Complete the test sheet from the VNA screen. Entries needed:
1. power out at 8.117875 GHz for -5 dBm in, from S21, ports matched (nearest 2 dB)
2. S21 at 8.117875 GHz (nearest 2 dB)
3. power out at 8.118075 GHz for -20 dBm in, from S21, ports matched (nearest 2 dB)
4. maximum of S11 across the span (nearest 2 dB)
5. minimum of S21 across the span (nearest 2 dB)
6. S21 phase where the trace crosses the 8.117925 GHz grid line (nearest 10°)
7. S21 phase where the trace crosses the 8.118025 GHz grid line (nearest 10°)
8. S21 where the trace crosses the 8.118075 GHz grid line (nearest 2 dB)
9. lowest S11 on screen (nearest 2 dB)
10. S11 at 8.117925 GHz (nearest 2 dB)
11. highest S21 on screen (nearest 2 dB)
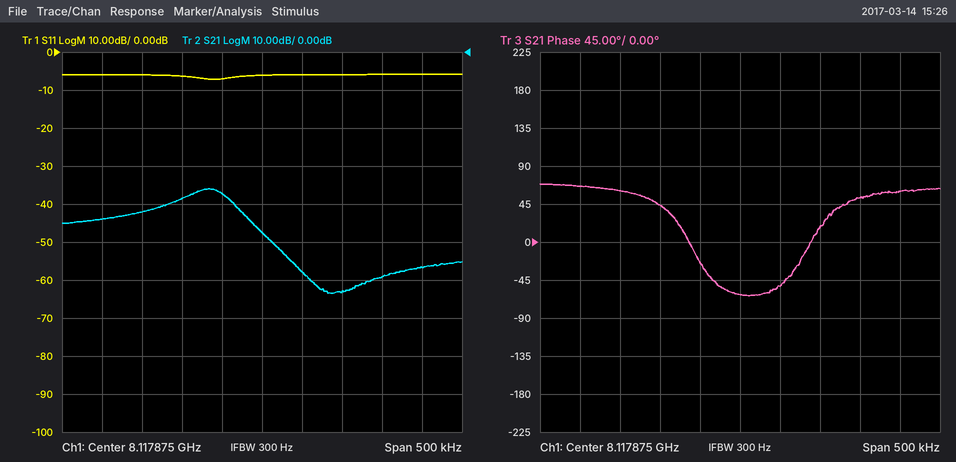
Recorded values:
-52 dBm
-48 dB
-76 dBm
-6 dB
-64 dB
-50°
50°
-56 dB
-8 dB
-6 dB
-36 dB
